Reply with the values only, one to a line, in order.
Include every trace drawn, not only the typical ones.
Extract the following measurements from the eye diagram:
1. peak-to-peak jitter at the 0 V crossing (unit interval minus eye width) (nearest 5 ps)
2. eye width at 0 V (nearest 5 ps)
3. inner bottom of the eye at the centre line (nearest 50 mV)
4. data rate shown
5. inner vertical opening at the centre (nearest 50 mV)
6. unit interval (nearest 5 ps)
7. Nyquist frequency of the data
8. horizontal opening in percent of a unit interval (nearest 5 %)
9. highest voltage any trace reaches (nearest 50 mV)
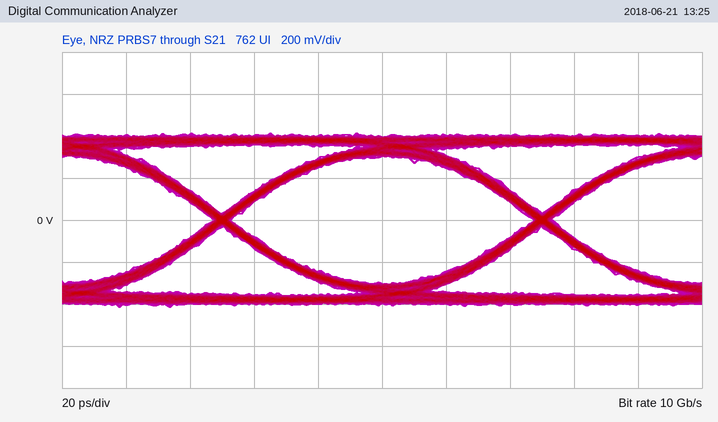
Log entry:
5 ps
95 ps
-300 mV
10 Gb/s
600 mV
100 ps
5 GHz
95 %
400 mV
